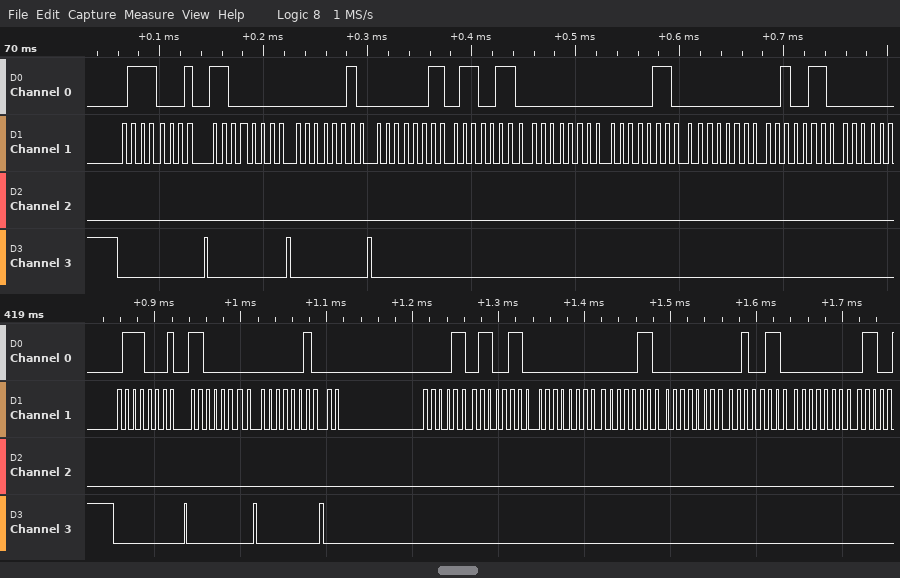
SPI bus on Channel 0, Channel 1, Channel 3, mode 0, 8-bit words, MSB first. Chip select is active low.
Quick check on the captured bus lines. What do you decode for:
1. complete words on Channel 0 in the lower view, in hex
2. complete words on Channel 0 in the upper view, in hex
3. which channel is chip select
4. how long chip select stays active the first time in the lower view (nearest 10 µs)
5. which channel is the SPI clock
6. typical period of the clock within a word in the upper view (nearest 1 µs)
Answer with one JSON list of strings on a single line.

["71, C0, 02, 03, 66, 00, 06, 00, 26, 00", "71, C0, 02, 03, 66, 00, 06, 00, 26", "Channel 3", "80 µs", "Channel 1", "9 µs"]
